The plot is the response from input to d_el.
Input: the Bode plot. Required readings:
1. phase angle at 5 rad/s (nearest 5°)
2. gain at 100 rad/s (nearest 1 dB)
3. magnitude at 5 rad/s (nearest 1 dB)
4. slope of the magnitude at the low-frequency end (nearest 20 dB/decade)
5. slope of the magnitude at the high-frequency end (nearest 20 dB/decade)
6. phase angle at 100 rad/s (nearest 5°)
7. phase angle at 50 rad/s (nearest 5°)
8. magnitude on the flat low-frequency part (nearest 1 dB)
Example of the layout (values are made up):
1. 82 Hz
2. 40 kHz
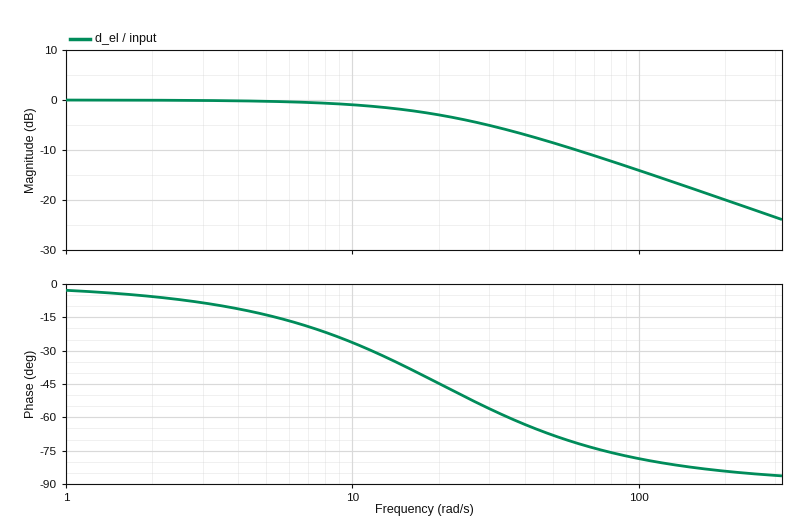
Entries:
1. -15°
2. -14 dB
3. 0 dB
4. 0 dB/decade
5. -20 dB/decade
6. -80°
7. -70°
8. 0 dB
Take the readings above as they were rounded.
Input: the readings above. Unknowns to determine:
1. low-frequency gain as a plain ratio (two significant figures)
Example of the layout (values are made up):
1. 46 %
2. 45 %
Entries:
1. 1.0
